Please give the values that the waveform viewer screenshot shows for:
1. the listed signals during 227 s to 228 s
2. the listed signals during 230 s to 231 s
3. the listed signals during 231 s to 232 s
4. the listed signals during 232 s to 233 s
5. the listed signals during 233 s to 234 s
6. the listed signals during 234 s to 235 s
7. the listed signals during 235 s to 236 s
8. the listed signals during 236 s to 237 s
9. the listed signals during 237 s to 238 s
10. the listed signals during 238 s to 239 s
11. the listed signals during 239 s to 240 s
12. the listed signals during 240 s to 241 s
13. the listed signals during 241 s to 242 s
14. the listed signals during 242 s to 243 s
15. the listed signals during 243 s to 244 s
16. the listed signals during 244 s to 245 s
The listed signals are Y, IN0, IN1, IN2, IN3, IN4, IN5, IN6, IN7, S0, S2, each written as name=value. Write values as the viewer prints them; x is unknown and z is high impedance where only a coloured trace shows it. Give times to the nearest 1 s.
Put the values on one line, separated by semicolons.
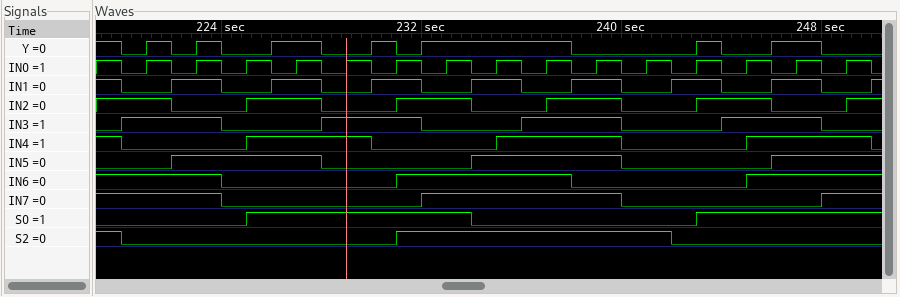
Y=1, IN0=1, IN1=1, IN2=1, IN3=0, IN4=1, IN5=1, IN6=0, IN7=0, S0=1, S2=0; Y=1, IN0=0, IN1=1, IN2=0, IN3=1, IN4=0, IN5=0, IN6=0, IN7=0, S0=1, S2=0; Y=0, IN0=1, IN1=1, IN2=1, IN3=1, IN4=0, IN5=0, IN6=1, IN7=0, S0=1, S2=1; Y=1, IN0=0, IN1=0, IN2=1, IN3=0, IN4=0, IN5=0, IN6=1, IN7=1, S0=1, S2=1; Y=1, IN0=1, IN1=0, IN2=1, IN3=0, IN4=0, IN5=0, IN6=1, IN7=1, S0=1, S2=1; Y=1, IN0=0, IN1=1, IN2=0, IN3=0, IN4=0, IN5=1, IN6=1, IN7=1, S0=0, S2=1; Y=1, IN0=1, IN1=1, IN2=0, IN3=0, IN4=1, IN5=1, IN6=1, IN7=1, S0=0, S2=1; Y=1, IN0=0, IN1=0, IN2=0, IN3=1, IN4=1, IN5=1, IN6=1, IN7=1, S0=0, S2=1; Y=1, IN0=1, IN1=0, IN2=1, IN3=1, IN4=1, IN5=1, IN6=1, IN7=1, S0=0, S2=1; Y=0, IN0=0, IN1=1, IN2=1, IN3=1, IN4=1, IN5=1, IN6=0, IN7=1, S0=0, S2=1; Y=0, IN0=1, IN1=1, IN2=1, IN3=1, IN4=1, IN5=1, IN6=0, IN7=1, S0=0, S2=1; Y=0, IN0=0, IN1=0, IN2=0, IN3=0, IN4=0, IN5=0, IN6=0, IN7=0, S0=0, S2=1; Y=0, IN0=1, IN1=0, IN2=0, IN3=0, IN4=0, IN5=0, IN6=0, IN7=0, S0=0, S2=1; Y=0, IN0=0, IN1=1, IN2=0, IN3=0, IN4=0, IN5=0, IN6=0, IN7=0, S0=0, S2=0; Y=1, IN0=1, IN1=1, IN2=1, IN3=0, IN4=0, IN5=0, IN6=0, IN7=0, S0=1, S2=0; Y=0, IN0=0, IN1=0, IN2=1, IN3=1, IN4=0, IN5=0, IN6=0, IN7=0, S0=1, S2=0
